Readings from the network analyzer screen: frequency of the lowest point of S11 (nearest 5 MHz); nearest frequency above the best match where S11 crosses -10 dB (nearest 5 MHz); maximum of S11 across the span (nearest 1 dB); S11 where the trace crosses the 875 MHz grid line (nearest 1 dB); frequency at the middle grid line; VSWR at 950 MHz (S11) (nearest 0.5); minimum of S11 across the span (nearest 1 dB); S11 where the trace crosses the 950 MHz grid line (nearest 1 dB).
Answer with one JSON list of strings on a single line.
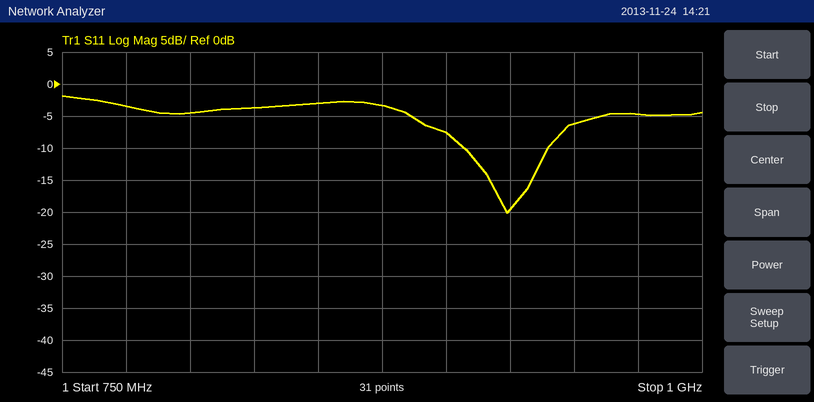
["925 MHz", "940 MHz", "-2 dB", "-3 dB", "875 MHz", "3.0", "-20 dB", "-6 dB"]
